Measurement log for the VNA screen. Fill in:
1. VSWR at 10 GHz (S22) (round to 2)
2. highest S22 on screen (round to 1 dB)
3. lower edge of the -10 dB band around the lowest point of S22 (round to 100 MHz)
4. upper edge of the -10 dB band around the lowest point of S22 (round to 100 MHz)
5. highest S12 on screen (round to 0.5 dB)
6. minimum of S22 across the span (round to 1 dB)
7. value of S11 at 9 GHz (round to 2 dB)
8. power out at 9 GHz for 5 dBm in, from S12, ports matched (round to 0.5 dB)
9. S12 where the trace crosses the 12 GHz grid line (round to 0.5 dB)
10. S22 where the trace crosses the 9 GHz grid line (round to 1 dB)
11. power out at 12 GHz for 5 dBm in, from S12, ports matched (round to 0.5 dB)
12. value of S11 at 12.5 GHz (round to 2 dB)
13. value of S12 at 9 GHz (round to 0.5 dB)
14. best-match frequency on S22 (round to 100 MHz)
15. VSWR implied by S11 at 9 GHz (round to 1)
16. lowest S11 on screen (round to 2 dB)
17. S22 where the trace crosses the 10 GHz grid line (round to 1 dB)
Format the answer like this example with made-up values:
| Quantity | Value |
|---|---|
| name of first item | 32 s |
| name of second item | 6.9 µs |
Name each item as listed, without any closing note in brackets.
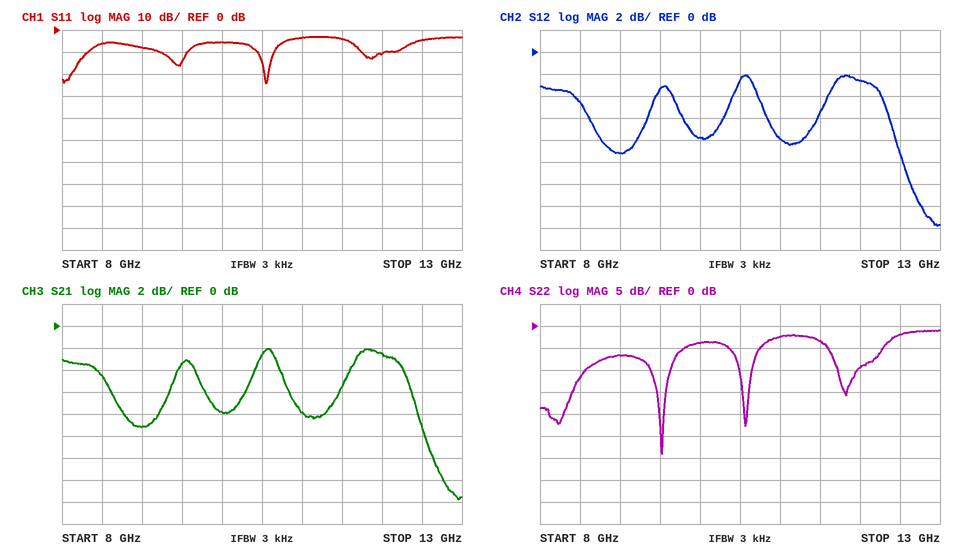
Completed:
| Quantity | Value |
|---|---|
| VSWR at 10 GHz (S22) | 4 |
| highest S22 on screen | -1 dB |
| lower edge of the -10 dB band around the lowest point of S22 | 9.4 GHz |
| upper edge of the -10 dB band around the lowest point of S22 | 9.6 GHz |
| highest S12 on screen | -2.0 dB |
| minimum of S22 across the span | -29 dB |
| value of S11 at 9 GHz | -8 dB |
| power out at 9 GHz for 5 dBm in, from S12, ports matched | -4.0 dBm |
| S12 where the trace crosses the 12 GHz grid line | -2.5 dB |
| S22 where the trace crosses the 9 GHz grid line | -7 dB |
| power out at 12 GHz for 5 dBm in, from S12, ports matched | 2.5 dBm |
| value of S11 at 12.5 GHz | -4 dB |
| value of S12 at 9 GHz | -9.0 dB |
| best-match frequency on S22 | 9.5 GHz |
| VSWR implied by S11 at 9 GHz | 2 |
| lowest S11 on screen | -24 dB |
| S22 where the trace crosses the 10 GHz grid line | -4 dB |
